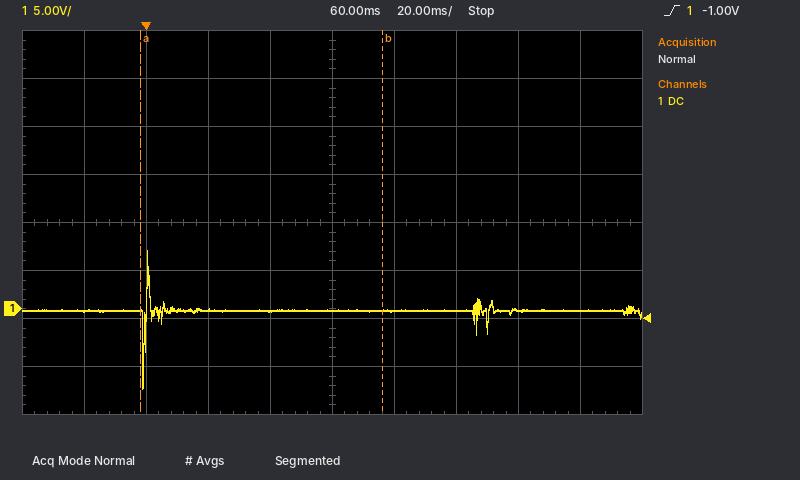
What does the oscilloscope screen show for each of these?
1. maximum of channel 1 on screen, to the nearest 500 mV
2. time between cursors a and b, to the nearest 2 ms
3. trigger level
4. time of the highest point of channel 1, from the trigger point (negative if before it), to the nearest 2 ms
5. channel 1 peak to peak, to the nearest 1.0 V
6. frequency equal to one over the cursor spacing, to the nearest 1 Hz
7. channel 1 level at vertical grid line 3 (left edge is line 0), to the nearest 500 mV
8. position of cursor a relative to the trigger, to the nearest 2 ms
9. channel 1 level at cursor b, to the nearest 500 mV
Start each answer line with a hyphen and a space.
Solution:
- 6.0 V
- 78 ms
- -1.00 V
- 0 ms
- 14.0 V
- 13 Hz
- 0.0 V
- -2 ms
- 0.0 V
